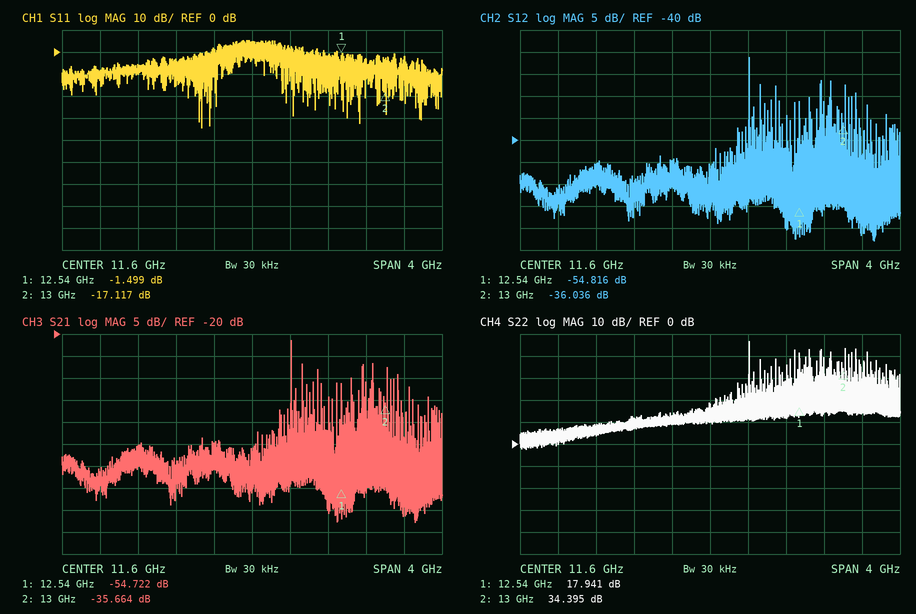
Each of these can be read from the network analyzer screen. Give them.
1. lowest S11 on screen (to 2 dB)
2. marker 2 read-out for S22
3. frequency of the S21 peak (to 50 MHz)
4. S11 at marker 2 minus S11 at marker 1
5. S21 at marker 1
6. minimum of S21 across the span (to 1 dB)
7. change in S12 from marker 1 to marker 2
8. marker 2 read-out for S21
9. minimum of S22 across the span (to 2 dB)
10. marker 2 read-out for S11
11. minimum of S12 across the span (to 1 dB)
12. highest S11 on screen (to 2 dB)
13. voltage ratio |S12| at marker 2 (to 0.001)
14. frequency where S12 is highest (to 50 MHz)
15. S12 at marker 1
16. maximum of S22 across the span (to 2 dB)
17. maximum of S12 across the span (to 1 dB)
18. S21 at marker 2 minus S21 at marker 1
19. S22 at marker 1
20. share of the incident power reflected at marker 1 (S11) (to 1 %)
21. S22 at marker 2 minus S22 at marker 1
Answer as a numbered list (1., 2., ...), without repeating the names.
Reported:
1. -34 dB
2. 34.395 dB
3. 12.00 GHz
4. -15.618 dB
5. -54.722 dB
6. -63 dB
7. 18.780 dB
8. -35.664 dB
9. -2 dB
10. -17.117 dB
11. -63 dB
12. 6 dB
13. 0.016
14. 12.00 GHz
15. -54.816 dB
16. 46 dB
17. -21 dB
18. 19.058 dB
19. 17.941 dB
20. 71 %
21. 16.454 dB
